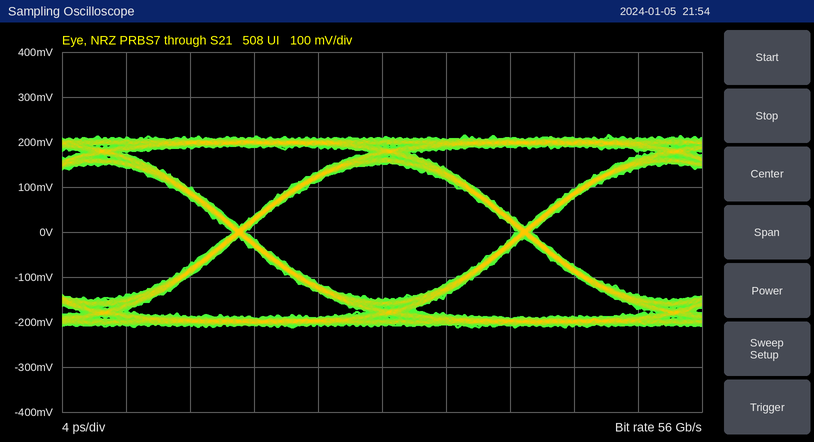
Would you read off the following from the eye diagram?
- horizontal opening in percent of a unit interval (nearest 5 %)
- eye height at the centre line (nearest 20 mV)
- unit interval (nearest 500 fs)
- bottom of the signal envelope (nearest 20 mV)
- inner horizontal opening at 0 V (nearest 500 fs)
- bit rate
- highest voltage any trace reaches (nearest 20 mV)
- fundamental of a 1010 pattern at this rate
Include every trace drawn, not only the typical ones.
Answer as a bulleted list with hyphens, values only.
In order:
- 95 %
- 300 mV
- 18.0 ps
- -220 mV
- 17.0 ps
- 56 Gb/s
- 220 mV
- 28 GHz
